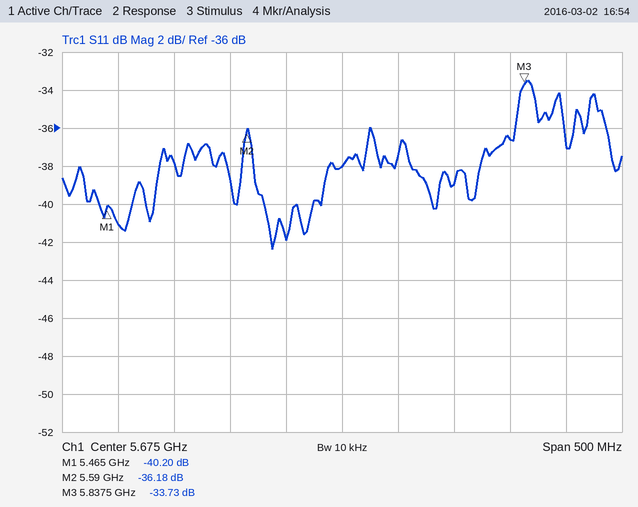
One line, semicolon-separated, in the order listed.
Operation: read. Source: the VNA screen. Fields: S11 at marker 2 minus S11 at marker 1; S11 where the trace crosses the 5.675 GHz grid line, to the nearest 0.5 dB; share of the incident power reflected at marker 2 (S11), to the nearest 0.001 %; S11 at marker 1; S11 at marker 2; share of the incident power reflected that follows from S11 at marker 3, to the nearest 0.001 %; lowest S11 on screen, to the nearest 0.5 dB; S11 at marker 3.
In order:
4.02 dB; -38.0 dB; 0.024 %; -40.20 dB; -36.18 dB; 0.042 %; -42.5 dB; -33.73 dB
